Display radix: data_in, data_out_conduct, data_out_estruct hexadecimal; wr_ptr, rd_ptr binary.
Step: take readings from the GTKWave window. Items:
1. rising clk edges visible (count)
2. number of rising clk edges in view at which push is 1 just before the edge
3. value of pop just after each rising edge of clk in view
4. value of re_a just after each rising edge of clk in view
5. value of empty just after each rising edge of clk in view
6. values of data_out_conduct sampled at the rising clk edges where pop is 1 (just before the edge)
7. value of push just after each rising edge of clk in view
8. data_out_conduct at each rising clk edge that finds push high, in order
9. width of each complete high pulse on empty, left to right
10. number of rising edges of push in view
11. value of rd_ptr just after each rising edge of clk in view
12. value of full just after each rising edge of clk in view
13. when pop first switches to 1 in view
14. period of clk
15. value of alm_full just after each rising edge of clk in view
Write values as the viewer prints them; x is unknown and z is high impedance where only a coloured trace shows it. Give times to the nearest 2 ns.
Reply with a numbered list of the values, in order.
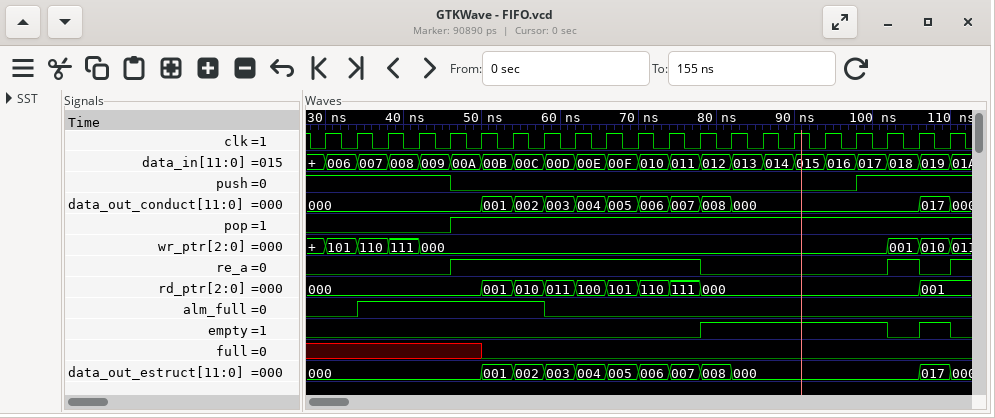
1. 21
2. 8
3. 0 0 0 0 1 1 1 1 1 1 1 1 1 1 1 1 1 1 1 1 1
4. 0 0 0 0 1 1 1 1 1 1 1 1 0 0 0 0 0 0 1 0 1
5. 0 0 0 0 0 0 0 0 0 0 0 0 1 1 1 1 1 1 0 1 0
6. 000, 001, 002, 003, 004, 005, 006, 007, 008, 000, 000, 000, 000, 000, 000, 017
7. 1 1 1 1 0 0 0 0 0 0 0 0 0 0 0 0 0 1 1 1 1
8. 000, 000, 000, 000, 000, 000, 000, 017
9. 24 ns, 4 ns
10. 1
11. 000, 000, 000, 000, 000, 001, 010, 011, 100, 101, 110, 111, 000, 000, 000, 000, 000, 000, 000, 001, 001
12. x x x x x 0 0 0 0 0 0 0 0 0 0 0 0 0 0 0 0
13. 46 ns
14. 4 ns
15. 0 1 1 1 1 1 1 0 0 0 0 0 0 0 0 0 0 0 0 0 0
